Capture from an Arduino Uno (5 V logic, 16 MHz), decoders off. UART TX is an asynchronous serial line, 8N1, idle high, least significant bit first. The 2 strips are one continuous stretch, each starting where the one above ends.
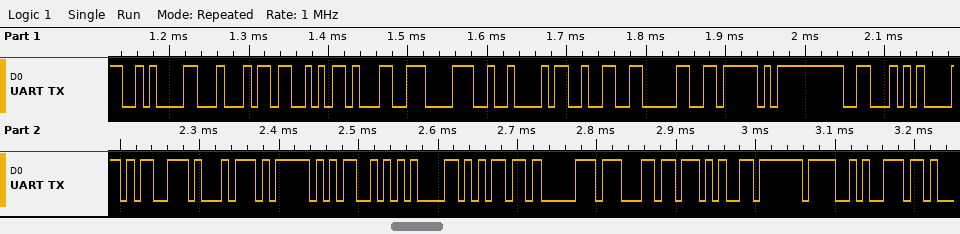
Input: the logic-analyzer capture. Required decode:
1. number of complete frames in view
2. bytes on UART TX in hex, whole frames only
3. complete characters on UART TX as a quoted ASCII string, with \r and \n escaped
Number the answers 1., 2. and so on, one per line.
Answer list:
1. 22
2. 0A 44 53 31 38 42 32 30 5F 46 61 73 74 5F 53 61 6D 70 6C 65 4F 6E
3. "\nDS18B20_Fast_SampleOn"
